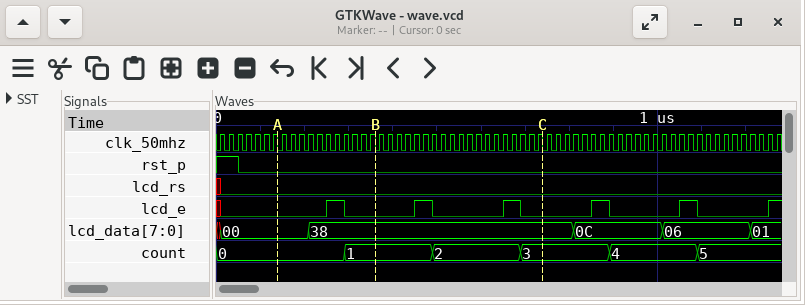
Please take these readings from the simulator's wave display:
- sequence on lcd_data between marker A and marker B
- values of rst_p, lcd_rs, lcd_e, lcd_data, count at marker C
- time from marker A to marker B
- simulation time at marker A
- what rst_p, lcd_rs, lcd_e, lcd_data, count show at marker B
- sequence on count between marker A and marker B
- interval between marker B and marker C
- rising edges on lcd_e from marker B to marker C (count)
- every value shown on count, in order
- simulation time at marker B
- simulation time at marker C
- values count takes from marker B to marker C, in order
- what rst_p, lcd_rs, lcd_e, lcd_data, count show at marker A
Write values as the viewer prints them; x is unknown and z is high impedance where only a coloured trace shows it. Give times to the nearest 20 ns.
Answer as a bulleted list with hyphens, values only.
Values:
- 00, 38
- rst_p=0, lcd_rs=0, lcd_e=0, lcd_data=38, count=3
- 220 ns
- 140 ns
- rst_p=0, lcd_rs=0, lcd_e=0, lcd_data=38, count=1
- 0, 1
- 380 ns
- 2
- 0, 1, 2, 3, 4, 5
- 360 ns
- 740 ns
- 1, 2, 3
- rst_p=0, lcd_rs=0, lcd_e=0, lcd_data=00, count=0
